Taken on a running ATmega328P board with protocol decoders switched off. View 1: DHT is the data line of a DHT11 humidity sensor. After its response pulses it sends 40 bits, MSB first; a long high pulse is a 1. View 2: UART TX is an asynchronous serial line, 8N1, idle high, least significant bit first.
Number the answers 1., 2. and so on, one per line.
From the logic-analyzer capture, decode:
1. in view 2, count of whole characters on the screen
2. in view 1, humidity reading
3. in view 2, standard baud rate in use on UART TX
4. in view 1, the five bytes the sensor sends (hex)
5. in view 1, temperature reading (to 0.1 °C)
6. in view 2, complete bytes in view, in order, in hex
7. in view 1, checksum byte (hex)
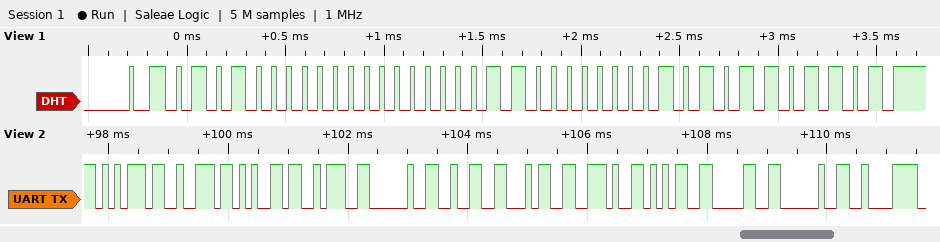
1. 12
2. 80 %
3. 9600 baud
4. 50 00 18 05 6D
5. 24.5 °C
6. 75 72 65 3A 20 32 34 2E 35 30 20 C2
7. 0x6D
